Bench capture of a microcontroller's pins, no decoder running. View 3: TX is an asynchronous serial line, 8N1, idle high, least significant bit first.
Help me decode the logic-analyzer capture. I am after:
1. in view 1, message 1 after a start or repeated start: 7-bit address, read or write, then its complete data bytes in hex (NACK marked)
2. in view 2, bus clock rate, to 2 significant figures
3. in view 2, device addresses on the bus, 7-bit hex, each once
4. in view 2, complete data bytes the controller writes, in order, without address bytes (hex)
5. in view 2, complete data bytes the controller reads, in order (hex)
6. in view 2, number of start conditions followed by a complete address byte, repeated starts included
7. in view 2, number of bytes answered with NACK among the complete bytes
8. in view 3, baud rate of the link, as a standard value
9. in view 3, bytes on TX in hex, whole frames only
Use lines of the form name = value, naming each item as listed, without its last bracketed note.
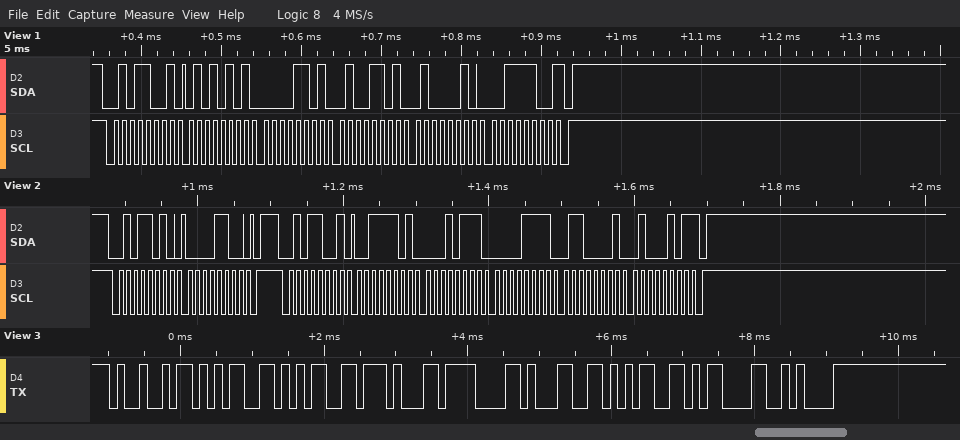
in view 1, message 1 after a start or repeated start: 7-bit address, read or write, then its complete data bytes in hex = 0x2C read: 55 0D 4D 42 3C NACK
in view 2, bus clock rate, to 2 significant figures = 100 kHz
in view 2, device addresses on the bus, 7-bit hex, each once = 0x2D 0x2C
in view 2, complete data bytes the controller writes, in order, without address bytes = 0C
in view 2, complete data bytes the controller reads, in order = 3D 17 0F 61 45
in view 2, number of start conditions followed by a complete address byte, repeated starts included = 2
in view 2, number of bytes answered with NACK among the complete bytes = 1
in view 3, baud rate of the link, as a standard value = 9600 baud
in view 3, bytes on TX in hex, whole frames only = 49 35 35 17 0F 31 35 0D 0A
